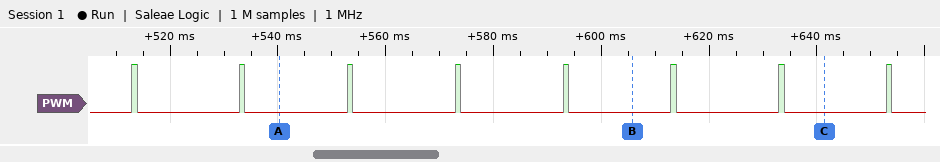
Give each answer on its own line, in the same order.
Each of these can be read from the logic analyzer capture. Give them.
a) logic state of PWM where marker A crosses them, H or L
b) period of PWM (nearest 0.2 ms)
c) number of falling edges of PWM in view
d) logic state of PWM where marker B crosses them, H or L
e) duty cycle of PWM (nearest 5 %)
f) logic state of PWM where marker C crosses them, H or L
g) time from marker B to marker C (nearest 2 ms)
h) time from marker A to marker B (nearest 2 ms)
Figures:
PWM=L
20 ms
8
PWM=L
5 %
PWM=L
36 ms
66 ms
